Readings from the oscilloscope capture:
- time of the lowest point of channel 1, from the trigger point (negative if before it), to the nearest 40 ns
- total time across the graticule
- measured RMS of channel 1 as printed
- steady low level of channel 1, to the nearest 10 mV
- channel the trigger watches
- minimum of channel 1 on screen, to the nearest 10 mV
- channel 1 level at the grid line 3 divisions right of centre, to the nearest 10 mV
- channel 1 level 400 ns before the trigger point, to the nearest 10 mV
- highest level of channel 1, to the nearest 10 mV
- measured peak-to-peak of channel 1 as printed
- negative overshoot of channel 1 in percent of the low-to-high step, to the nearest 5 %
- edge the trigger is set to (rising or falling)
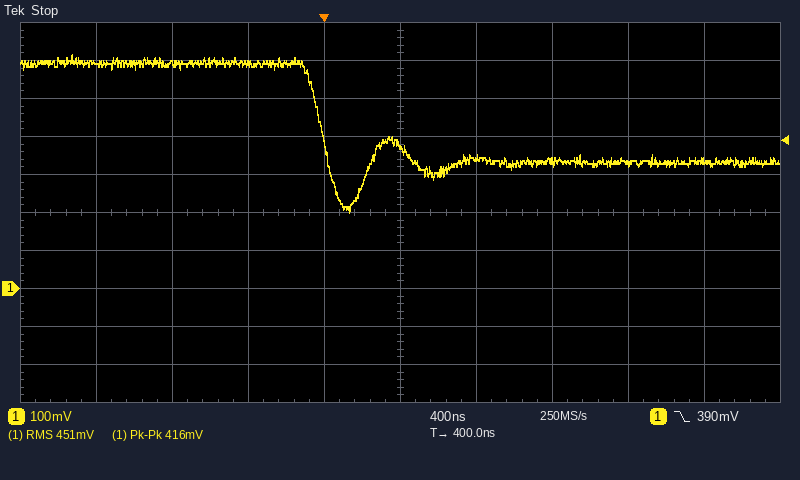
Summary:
+120 ns
4 µs
451 mV
330 mV
channel 1
200 mV
330 mV
590 mV
620 mV
416 mV
50 %
falling
